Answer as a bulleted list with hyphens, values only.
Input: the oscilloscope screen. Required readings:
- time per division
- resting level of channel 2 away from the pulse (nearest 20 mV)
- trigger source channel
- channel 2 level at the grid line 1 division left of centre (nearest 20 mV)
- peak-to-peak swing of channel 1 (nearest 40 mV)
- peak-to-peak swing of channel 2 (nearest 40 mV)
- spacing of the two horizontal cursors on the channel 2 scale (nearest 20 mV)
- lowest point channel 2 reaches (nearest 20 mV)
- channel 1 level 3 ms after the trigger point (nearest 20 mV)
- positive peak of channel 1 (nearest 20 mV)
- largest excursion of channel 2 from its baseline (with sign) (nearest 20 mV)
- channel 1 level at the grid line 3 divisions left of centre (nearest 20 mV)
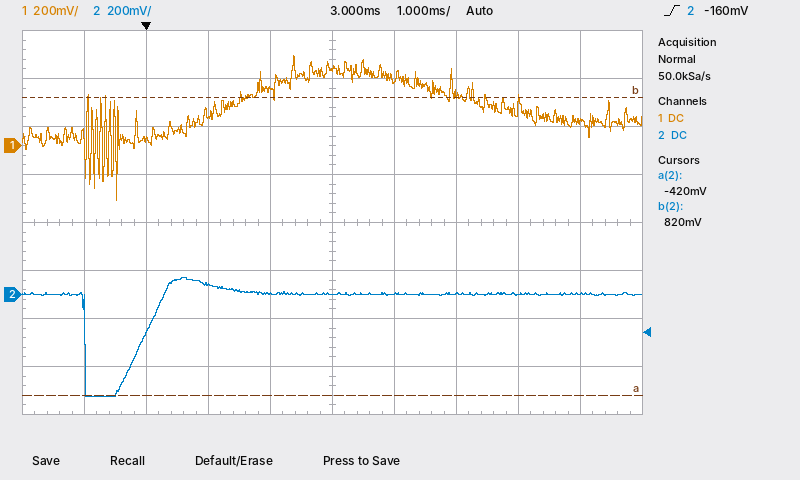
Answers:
- 1 ms
- 0 mV
- channel 2
- 0 mV
- 600 mV
- 480 mV
- 1.24 V
- -420 mV
- 320 mV
- 380 mV
- -420 mV
- 20 mV
